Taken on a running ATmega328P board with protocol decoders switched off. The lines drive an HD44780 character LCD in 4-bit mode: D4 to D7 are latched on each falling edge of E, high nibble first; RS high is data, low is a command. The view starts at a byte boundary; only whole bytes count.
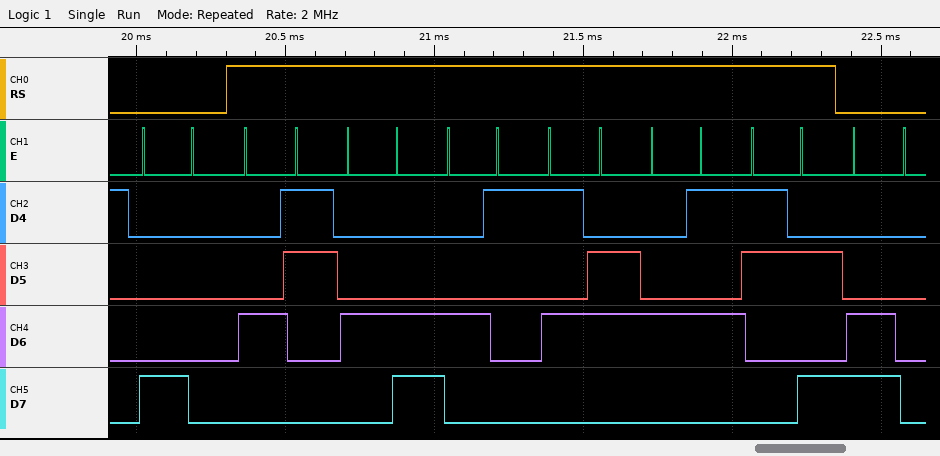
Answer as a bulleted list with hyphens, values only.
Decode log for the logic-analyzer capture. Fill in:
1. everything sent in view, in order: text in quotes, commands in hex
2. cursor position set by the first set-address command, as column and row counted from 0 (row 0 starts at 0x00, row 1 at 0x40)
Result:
- 0x80 "CLAVE:" 0xC0
- column 0, row 0
